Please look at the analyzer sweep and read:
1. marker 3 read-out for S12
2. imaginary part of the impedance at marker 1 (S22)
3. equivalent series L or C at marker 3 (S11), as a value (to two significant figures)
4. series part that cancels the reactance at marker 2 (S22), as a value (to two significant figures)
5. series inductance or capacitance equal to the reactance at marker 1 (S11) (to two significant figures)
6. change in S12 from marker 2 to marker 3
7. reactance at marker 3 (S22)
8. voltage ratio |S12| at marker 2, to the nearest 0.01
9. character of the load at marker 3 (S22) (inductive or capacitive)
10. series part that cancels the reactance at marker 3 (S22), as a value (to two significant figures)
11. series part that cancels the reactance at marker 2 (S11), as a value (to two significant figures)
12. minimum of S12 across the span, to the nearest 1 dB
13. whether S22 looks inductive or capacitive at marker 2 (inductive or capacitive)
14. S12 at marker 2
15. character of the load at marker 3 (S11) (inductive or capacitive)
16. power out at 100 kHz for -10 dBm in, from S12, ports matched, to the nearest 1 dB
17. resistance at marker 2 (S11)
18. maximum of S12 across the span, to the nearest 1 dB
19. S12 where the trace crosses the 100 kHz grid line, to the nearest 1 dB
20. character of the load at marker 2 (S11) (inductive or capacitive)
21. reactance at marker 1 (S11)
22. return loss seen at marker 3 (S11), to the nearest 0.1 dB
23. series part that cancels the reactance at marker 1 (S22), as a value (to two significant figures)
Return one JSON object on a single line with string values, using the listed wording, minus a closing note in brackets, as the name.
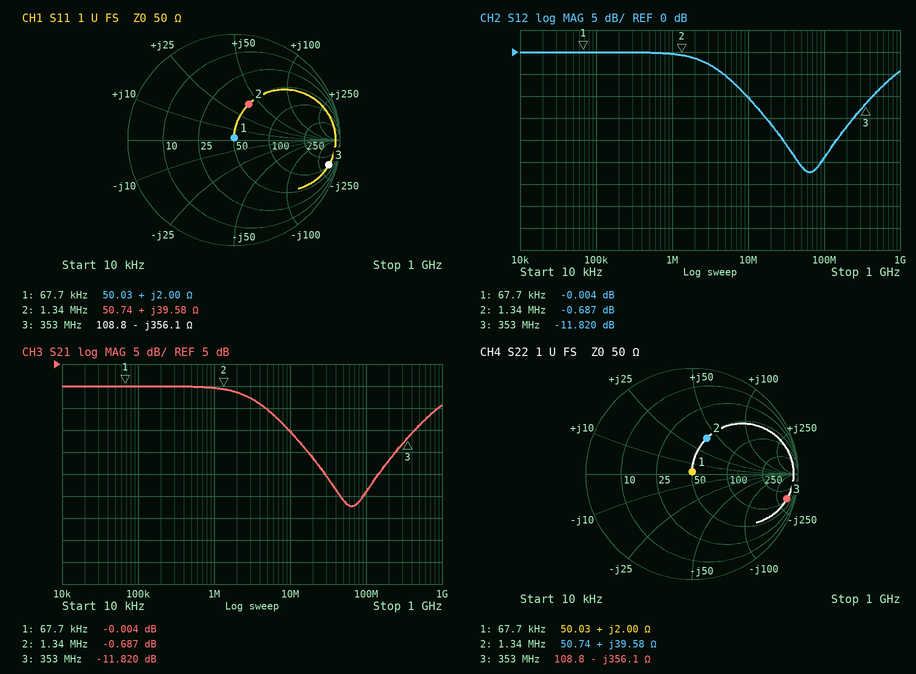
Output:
{"marker 3 read-out for S12": "-11.820 dB", "imaginary part of the impedance at marker 1": "+2.00 Ω", "equivalent series L or C at marker 3 (S11), as a value": "1.3 pF", "series part that cancels the reactance at marker 2 (S22), as a value": "3.0 nF", "series inductance or capacitance equal to the reactance at marker 1 (S11)": "4.7 µH", "change in S12 from marker 2 to marker 3": "-11.133 dB", "reactance at marker 3": "-356.1 Ω", "voltage ratio |S12| at marker 2, to the nearest 0.01": "0.92", "character of the load at marker 3 (S22)": "capacitive", "series part that cancels the reactance at marker 3 (S22), as a value": "160 nH", "series part that cancels the reactance at marker 2 (S11), as a value": "3.0 nF", "minimum of S12 across the span, to the nearest 1 dB": "-27 dB", "whether S22 looks inductive or capacitive at marker 2": "inductive", "S12 at marker 2": "-0.687 dB", "character of the load at marker 3 (S11)": "capacitive", "power out at 100 kHz for -10 dBm in, from S12, ports matched, to the nearest 1 dB": "-10 dBm", "resistance at marker 2": "50.74 Ω", "maximum of S12 across the span, to the nearest 1 dB": "0 dB", "S12 where the trace crosses the 100 kHz grid line, to the nearest 1 dB": "0 dB", "character of the load at marker 2 (S11)": "inductive", "reactance at marker 1": "+2.00 Ω", "return loss seen at marker 3 (S11), to the nearest 0.1 dB": "0.7 dB", "series part that cancels the reactance at marker 1 (S22), as a value": "1.2 µF"}
